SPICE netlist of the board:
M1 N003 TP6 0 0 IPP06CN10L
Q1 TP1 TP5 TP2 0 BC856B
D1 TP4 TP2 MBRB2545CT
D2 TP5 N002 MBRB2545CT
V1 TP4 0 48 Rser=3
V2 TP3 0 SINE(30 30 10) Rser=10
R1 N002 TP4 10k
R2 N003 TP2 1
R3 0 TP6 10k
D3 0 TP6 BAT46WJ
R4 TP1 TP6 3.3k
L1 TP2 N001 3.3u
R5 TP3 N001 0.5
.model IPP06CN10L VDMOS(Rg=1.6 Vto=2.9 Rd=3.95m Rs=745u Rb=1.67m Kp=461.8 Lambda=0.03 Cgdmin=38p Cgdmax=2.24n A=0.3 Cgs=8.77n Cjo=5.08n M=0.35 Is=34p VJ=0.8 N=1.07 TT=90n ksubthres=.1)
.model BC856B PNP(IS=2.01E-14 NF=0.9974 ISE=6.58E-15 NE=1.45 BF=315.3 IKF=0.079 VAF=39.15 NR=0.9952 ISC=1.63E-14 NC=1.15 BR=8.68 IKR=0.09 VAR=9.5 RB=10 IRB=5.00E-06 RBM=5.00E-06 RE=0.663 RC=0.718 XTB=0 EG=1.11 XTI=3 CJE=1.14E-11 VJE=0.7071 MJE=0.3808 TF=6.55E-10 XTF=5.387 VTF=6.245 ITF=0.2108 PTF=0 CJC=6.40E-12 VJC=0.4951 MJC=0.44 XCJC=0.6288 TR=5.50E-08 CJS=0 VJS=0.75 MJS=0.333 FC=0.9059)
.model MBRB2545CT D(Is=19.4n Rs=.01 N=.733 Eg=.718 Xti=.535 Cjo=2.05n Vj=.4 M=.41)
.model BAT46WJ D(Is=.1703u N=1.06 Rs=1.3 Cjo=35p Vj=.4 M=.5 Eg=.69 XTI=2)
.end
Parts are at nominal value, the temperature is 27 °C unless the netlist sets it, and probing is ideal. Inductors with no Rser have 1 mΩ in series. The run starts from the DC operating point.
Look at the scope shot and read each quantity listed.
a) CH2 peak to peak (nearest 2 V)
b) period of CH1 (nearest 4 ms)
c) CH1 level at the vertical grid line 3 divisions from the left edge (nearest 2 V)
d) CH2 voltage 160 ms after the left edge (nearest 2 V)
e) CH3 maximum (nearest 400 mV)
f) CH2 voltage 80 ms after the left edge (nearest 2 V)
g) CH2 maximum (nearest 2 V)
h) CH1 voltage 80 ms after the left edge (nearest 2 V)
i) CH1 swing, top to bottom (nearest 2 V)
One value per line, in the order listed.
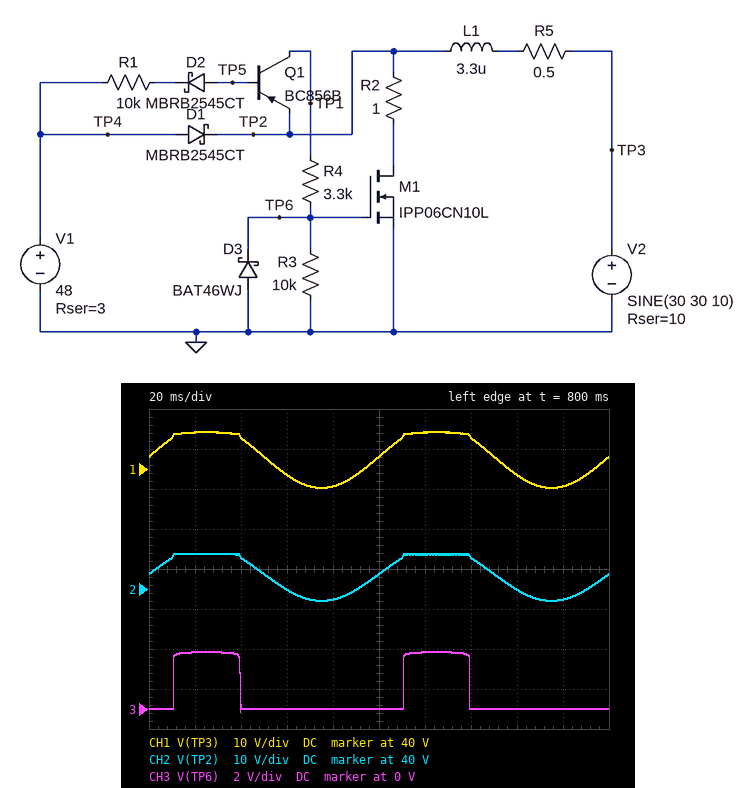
12 V
100 ms
38 V
40 V
2.8 V
38 V
48 V
36 V
14 V
